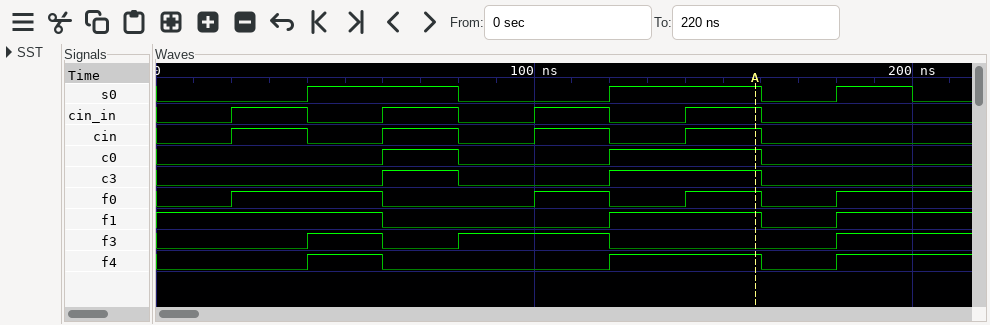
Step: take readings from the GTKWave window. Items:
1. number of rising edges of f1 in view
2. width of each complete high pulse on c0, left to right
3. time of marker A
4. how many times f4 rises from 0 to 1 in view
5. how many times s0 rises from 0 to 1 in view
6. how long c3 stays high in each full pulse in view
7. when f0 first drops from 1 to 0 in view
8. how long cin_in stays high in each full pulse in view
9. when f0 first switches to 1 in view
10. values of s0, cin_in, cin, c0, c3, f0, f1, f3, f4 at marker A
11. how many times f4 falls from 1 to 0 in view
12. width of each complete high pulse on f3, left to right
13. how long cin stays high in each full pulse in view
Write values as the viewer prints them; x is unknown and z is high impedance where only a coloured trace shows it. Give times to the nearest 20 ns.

2
20 ns, 40 ns
160 ns
3
3
20 ns, 40 ns
60 ns
20 ns, 20 ns, 20 ns, 20 ns
20 ns
s0=1, cin_in=1, cin=1, c0=1, c3=1, f0=1, f1=1, f3=0, f4=1
2
20 ns, 40 ns
20 ns, 20 ns, 20 ns, 20 ns
